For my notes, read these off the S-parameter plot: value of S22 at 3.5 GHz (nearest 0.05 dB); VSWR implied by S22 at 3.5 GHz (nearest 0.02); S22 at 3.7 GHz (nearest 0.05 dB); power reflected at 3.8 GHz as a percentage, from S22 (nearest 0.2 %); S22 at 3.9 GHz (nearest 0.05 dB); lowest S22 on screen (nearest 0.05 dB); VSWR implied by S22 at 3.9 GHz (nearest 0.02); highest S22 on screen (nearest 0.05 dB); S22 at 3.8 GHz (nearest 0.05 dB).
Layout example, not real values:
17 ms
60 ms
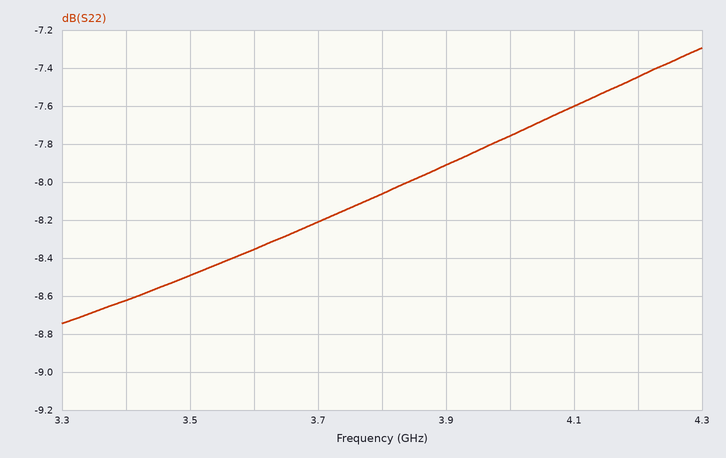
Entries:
-8.50 dB
2.20
-8.20 dB
15.6 %
-7.90 dB
-8.75 dB
2.34
-7.30 dB
-8.05 dB
